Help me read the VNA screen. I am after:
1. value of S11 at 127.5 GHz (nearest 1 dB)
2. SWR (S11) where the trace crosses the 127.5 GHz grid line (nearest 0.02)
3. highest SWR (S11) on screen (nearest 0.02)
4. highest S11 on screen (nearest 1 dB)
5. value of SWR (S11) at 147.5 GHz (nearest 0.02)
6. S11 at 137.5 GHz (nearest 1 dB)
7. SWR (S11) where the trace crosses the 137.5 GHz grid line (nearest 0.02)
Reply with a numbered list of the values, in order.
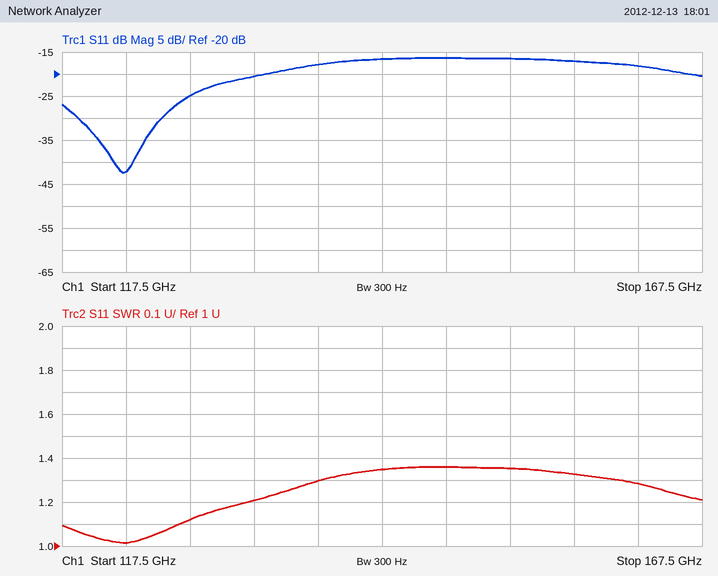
1. -25 dB
2. 1.12
3. 1.36
4. -16 dB
5. 1.36
6. -18 dB
7. 1.30
